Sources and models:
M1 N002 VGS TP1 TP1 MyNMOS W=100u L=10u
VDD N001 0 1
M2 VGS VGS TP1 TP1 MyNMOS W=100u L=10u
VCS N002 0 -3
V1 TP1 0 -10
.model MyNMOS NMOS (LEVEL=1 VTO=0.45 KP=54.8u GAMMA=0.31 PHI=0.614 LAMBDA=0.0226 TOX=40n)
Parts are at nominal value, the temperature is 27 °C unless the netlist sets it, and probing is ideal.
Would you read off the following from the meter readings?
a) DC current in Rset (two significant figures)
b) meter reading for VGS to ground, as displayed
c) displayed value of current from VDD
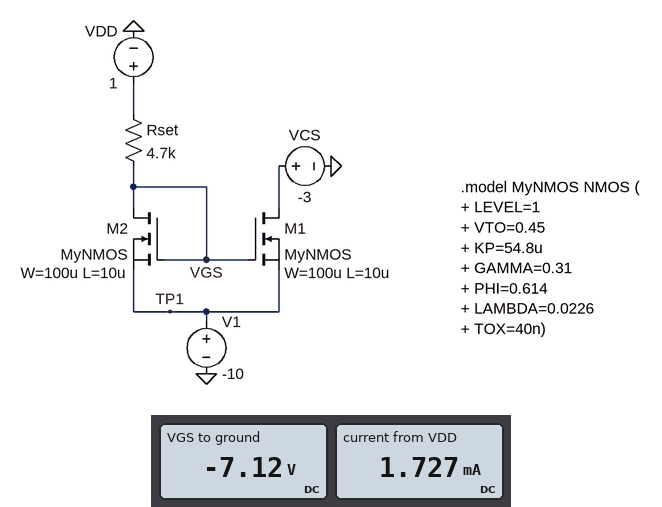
1.7 mA
-7.12 V
1.727 mA
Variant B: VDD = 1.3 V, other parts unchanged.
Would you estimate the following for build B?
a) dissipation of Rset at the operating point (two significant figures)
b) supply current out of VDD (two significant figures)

15 mW
1.8 mA
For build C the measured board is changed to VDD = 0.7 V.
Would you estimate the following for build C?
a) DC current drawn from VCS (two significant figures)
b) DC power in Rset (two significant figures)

1.8 mA
13 mW
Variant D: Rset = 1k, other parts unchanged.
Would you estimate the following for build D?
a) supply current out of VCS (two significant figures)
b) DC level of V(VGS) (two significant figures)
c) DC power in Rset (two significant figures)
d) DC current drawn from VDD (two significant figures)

6.3 mA
-5.1 V
37 mW
6.1 mA
